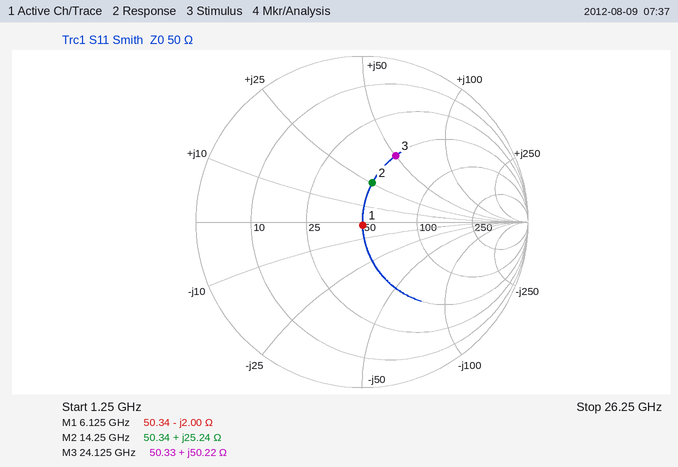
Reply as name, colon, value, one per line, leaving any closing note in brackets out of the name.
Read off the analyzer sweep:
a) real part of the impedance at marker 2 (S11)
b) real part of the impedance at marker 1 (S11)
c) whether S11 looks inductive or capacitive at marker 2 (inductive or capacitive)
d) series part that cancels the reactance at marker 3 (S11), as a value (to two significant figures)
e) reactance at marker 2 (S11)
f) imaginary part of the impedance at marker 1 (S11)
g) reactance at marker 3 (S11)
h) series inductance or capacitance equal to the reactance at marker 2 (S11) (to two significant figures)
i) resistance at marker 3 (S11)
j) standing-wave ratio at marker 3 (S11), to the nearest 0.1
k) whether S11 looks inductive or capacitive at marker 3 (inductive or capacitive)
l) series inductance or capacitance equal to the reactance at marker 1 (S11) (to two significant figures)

real part of the impedance at marker 2: 50.34 Ω
real part of the impedance at marker 1: 50.34 Ω
whether S11 looks inductive or capacitive at marker 2: inductive
series part that cancels the reactance at marker 3 (S11), as a value: 130 fF
reactance at marker 2: +25.24 Ω
imaginary part of the impedance at marker 1: -2.00 Ω
reactance at marker 3: +50.22 Ω
series inductance or capacitance equal to the reactance at marker 2 (S11): 280 pH
resistance at marker 3: 50.33 Ω
standing-wave ratio at marker 3 (S11), to the nearest 0.1: 2.6
whether S11 looks inductive or capacitive at marker 3: inductive
series inductance or capacitance equal to the reactance at marker 1 (S11): 13 pF
